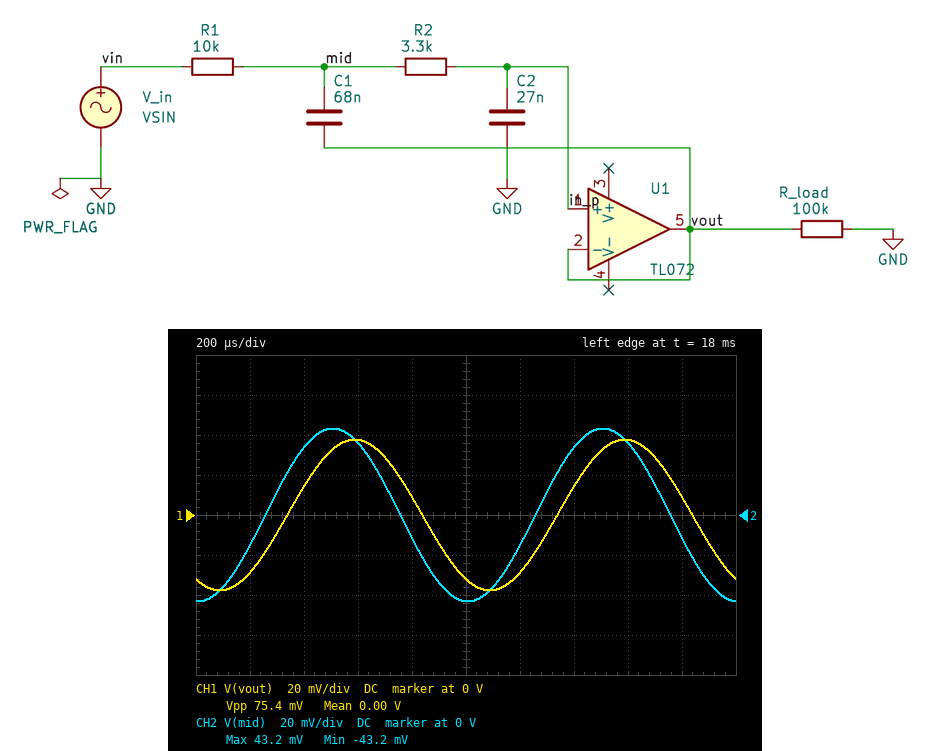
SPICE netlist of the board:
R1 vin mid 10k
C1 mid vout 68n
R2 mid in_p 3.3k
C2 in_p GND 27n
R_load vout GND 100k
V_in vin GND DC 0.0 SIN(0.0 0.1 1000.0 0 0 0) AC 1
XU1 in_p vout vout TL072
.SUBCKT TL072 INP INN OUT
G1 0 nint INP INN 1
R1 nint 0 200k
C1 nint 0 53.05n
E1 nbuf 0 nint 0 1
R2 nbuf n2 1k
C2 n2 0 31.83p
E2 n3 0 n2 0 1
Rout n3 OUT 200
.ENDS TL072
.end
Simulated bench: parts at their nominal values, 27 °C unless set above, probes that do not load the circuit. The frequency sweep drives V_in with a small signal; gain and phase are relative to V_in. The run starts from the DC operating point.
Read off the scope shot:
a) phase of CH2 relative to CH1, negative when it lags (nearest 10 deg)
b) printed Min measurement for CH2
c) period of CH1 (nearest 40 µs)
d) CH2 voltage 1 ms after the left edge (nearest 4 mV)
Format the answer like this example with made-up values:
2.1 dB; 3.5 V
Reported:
30 deg; -43.2 mV; 1.00 ms; -44 mV
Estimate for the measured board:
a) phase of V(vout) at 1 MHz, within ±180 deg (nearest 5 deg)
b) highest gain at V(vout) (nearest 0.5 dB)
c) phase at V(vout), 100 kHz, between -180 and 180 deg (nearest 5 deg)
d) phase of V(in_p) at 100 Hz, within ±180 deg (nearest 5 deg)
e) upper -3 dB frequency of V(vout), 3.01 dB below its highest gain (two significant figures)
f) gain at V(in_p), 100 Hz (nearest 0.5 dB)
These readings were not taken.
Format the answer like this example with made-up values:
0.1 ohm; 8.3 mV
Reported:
80 deg; 0 dB; 90 deg; -15 deg; 630 Hz; 0 dB
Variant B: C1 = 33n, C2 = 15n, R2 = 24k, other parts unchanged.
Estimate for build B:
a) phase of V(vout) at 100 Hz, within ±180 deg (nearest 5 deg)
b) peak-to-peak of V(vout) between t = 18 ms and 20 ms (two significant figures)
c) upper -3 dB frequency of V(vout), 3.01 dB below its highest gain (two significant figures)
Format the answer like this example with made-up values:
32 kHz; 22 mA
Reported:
-20 deg; 41 mV; 440 Hz
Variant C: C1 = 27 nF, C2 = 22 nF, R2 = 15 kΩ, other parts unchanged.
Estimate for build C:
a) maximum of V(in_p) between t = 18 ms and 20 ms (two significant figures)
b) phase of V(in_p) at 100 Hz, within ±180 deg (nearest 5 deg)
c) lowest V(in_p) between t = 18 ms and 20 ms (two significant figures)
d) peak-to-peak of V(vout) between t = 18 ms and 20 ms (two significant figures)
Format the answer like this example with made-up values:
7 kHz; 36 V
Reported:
23 mV; -20 deg; -23 mV; 47 mV
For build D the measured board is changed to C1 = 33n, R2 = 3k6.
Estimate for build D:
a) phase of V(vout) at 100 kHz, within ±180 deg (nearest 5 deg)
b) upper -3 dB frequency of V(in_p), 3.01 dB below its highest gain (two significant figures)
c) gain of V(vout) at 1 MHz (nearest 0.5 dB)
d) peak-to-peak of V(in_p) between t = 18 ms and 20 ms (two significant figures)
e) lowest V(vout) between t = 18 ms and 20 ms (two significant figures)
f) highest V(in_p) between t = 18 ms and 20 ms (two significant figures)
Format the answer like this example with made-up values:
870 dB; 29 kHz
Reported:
95 deg; 550 Hz; -43.5 dB; 86 mV; -43 mV; 43 mV
